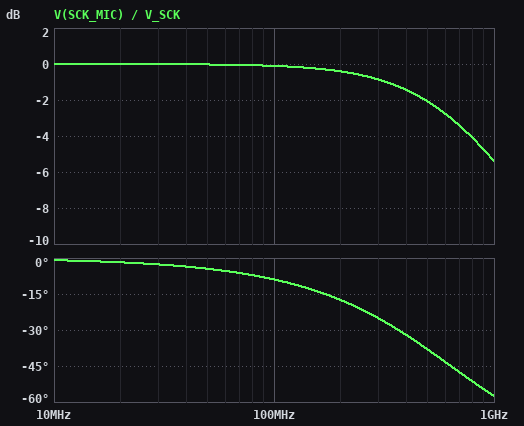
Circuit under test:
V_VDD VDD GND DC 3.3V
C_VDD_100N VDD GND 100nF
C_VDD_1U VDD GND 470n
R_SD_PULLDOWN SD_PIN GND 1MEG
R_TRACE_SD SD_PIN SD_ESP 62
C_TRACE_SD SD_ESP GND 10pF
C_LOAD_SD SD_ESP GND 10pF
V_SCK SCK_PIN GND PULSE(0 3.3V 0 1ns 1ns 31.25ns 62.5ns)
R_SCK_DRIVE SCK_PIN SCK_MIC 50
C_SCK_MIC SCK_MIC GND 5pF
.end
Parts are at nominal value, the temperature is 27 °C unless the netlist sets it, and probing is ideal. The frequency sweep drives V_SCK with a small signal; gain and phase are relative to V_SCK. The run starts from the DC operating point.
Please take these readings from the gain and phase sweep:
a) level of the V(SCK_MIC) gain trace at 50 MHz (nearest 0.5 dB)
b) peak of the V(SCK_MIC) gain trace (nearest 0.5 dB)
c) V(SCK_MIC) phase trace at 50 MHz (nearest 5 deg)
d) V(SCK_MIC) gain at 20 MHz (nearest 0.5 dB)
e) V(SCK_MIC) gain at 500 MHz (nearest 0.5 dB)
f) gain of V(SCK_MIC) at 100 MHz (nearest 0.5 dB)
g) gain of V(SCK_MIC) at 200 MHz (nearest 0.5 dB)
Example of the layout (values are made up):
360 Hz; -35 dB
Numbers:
0 dB; 0 dB; -5 deg; 0 dB; -2.0 dB; 0 dB; -0.5 dB
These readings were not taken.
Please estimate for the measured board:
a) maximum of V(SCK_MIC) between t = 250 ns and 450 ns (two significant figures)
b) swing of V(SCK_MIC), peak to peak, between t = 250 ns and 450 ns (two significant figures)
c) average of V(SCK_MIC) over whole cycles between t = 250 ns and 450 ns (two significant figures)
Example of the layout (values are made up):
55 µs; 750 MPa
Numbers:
3.3 V; 3.3 V; 1.7 V
